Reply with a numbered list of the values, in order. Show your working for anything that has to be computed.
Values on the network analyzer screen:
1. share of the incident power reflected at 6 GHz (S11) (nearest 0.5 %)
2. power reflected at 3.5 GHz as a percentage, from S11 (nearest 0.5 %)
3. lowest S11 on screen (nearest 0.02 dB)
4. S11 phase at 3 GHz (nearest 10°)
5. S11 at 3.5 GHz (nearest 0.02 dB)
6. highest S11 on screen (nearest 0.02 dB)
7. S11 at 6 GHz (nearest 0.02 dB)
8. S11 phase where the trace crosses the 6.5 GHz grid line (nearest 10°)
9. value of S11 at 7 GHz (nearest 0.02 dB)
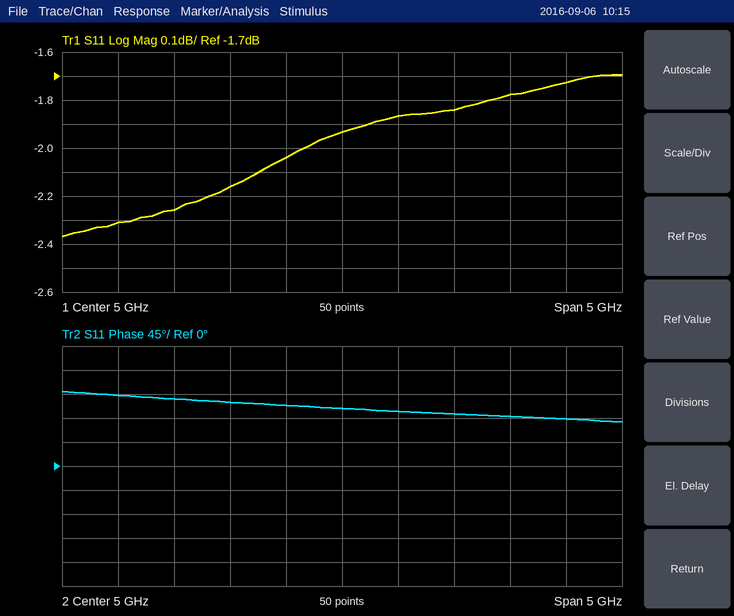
1. 10^(-1.84/10) ≈ 65.5 %
2. 10^(-2.26/10) ≈ 59.4 %, so 59.5 % to the nearest 0.5 %
3. -2.36 dB
4. 130°
5. -2.26 dB
6. -1.70 dB
7. -1.84 dB
8. 90°
9. -1.72 dB
